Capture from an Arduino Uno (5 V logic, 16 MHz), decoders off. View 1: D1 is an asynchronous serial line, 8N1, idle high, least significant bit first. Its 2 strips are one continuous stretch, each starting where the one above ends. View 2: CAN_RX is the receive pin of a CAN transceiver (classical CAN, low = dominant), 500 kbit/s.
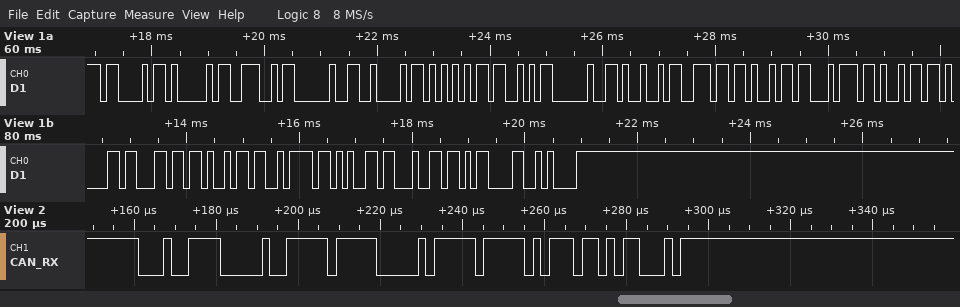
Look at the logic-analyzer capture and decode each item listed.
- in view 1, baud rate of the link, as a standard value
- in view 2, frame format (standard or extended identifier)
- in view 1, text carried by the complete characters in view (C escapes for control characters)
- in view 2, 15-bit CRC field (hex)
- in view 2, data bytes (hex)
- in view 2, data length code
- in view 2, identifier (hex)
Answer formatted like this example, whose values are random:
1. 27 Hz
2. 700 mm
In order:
1. 9600 baud
2. standard
3. "CAN BUS Initialized\r\n"
4. 0x3B58
5. FF 07 FF
6. 3
7. 0x13C
